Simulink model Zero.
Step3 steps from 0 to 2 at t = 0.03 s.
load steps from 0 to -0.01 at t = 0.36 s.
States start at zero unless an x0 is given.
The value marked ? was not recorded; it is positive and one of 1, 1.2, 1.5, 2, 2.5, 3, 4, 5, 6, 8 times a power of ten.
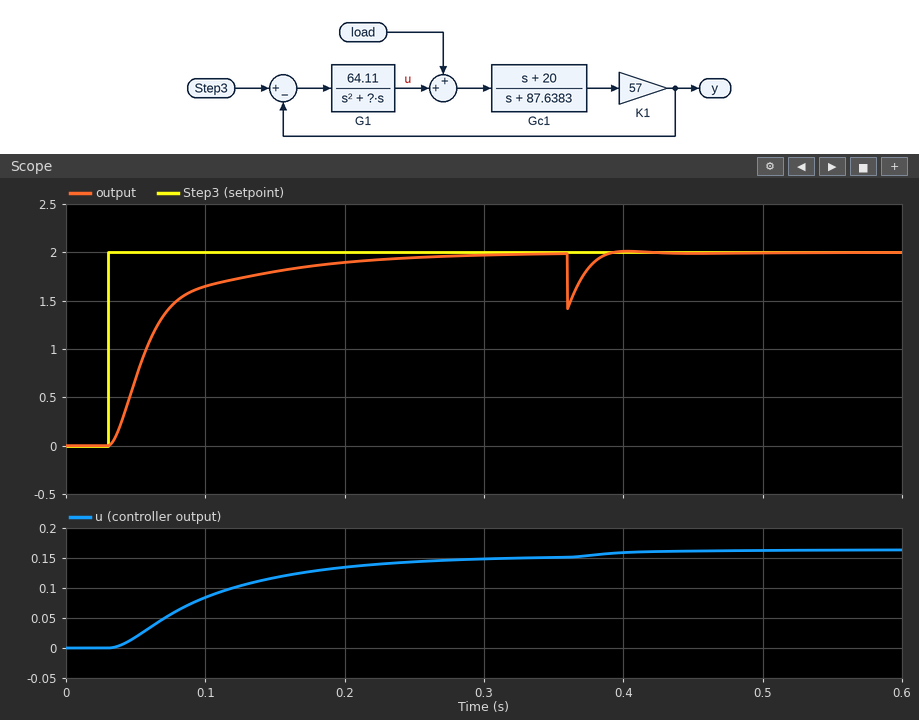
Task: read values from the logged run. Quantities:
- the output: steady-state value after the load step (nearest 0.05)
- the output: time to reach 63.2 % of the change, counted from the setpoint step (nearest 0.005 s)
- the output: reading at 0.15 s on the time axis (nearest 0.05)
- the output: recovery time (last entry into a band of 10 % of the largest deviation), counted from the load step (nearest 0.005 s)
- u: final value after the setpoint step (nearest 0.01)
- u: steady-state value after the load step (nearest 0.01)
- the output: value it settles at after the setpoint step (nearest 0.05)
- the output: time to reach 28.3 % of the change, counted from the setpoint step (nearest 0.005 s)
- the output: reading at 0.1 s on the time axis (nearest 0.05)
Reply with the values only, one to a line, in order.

2.00
0.035 s
1.80
0.025 s
0.15
0.16
2.00
0.015 s
1.65
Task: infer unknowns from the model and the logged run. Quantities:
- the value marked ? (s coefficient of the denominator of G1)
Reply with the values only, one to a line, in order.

40
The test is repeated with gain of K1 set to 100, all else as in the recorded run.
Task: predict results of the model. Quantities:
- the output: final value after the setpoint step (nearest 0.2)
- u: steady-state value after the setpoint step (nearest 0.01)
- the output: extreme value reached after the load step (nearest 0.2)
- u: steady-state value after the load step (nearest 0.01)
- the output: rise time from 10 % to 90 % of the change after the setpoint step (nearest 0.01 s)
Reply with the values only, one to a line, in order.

2.0
0.09
1.0
0.10
0.03 s
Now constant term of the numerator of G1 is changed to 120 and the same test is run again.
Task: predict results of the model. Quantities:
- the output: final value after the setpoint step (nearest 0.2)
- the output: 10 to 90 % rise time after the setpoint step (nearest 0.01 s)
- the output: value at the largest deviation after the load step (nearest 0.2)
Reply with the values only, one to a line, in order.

2.0
0.03 s
1.4
